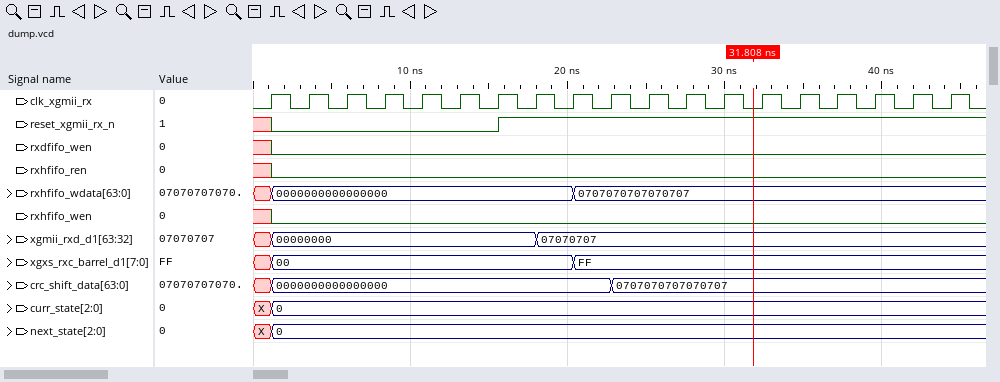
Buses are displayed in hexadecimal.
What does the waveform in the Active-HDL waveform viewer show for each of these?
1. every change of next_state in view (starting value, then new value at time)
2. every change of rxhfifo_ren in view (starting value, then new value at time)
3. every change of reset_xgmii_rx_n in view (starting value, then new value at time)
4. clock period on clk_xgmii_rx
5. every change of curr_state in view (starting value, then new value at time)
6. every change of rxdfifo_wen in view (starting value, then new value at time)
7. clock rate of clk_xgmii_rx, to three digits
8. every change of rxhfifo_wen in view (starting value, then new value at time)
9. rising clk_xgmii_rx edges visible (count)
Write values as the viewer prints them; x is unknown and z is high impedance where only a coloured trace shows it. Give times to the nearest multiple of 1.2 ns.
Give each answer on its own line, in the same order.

X, 0 at 1.2 ns
x, 0 at 1.2 ns
x, 0 at 1.2 ns, 1 at 15.6 ns
2.4 ns
X, 0 at 1.2 ns
x, 0 at 1.2 ns
417 MHz
x, 0 at 1.2 ns
19
